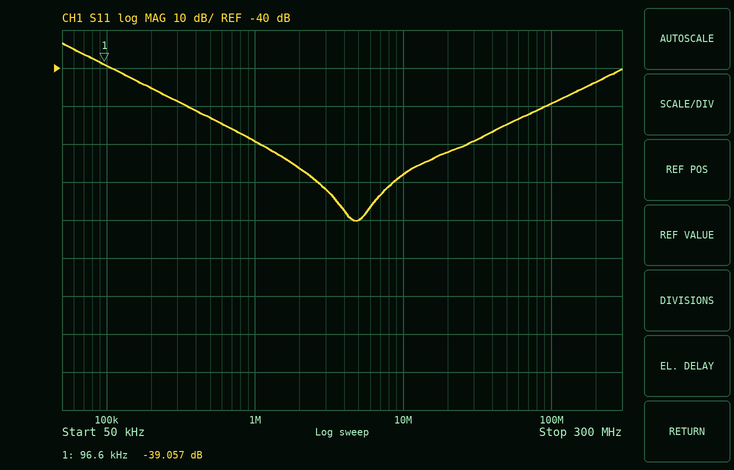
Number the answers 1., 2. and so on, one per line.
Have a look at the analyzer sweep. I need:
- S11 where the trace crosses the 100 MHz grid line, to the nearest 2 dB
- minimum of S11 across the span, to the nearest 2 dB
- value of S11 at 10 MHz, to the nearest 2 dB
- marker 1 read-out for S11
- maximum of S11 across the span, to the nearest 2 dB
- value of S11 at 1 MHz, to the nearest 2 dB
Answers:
1. -50 dB
2. -80 dB
3. -68 dB
4. -39.057 dB
5. -34 dB
6. -60 dB
